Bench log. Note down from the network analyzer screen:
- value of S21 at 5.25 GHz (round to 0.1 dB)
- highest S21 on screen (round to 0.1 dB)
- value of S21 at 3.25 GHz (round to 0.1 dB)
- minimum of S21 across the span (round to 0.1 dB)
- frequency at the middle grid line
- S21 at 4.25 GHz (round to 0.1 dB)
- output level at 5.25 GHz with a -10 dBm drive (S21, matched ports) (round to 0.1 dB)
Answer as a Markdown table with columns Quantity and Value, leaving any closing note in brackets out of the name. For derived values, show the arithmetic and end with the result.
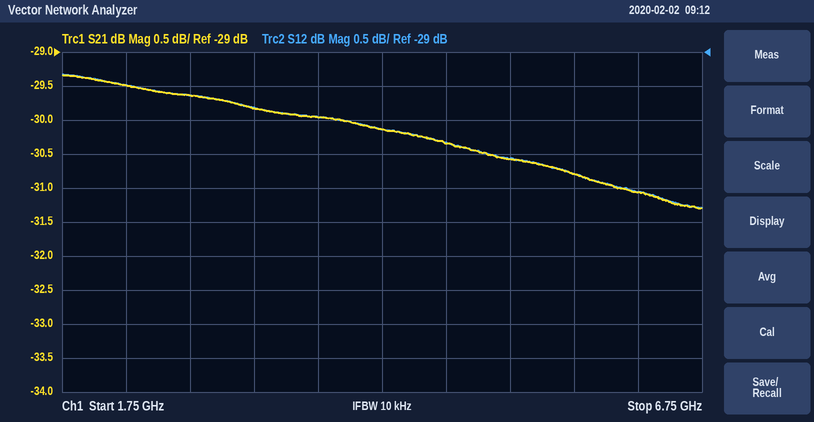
| Quantity | Value |
|---|---|
| value of S21 at 5.25 GHz | -30.6 dB |
| highest S21 on screen | -29.3 dB |
| value of S21 at 3.25 GHz | -29.8 dB |
| minimum of S21 across the span | -31.3 dB |
| frequency at the middle grid line | 4.25 GHz |
| S21 at 4.25 GHz | -30.1 dB |
| output level at 5.25 GHz with a -10 dBm drive (S21, matched ports) | -10 dBm + (-30.6 dB) = -40.6 dBm |
